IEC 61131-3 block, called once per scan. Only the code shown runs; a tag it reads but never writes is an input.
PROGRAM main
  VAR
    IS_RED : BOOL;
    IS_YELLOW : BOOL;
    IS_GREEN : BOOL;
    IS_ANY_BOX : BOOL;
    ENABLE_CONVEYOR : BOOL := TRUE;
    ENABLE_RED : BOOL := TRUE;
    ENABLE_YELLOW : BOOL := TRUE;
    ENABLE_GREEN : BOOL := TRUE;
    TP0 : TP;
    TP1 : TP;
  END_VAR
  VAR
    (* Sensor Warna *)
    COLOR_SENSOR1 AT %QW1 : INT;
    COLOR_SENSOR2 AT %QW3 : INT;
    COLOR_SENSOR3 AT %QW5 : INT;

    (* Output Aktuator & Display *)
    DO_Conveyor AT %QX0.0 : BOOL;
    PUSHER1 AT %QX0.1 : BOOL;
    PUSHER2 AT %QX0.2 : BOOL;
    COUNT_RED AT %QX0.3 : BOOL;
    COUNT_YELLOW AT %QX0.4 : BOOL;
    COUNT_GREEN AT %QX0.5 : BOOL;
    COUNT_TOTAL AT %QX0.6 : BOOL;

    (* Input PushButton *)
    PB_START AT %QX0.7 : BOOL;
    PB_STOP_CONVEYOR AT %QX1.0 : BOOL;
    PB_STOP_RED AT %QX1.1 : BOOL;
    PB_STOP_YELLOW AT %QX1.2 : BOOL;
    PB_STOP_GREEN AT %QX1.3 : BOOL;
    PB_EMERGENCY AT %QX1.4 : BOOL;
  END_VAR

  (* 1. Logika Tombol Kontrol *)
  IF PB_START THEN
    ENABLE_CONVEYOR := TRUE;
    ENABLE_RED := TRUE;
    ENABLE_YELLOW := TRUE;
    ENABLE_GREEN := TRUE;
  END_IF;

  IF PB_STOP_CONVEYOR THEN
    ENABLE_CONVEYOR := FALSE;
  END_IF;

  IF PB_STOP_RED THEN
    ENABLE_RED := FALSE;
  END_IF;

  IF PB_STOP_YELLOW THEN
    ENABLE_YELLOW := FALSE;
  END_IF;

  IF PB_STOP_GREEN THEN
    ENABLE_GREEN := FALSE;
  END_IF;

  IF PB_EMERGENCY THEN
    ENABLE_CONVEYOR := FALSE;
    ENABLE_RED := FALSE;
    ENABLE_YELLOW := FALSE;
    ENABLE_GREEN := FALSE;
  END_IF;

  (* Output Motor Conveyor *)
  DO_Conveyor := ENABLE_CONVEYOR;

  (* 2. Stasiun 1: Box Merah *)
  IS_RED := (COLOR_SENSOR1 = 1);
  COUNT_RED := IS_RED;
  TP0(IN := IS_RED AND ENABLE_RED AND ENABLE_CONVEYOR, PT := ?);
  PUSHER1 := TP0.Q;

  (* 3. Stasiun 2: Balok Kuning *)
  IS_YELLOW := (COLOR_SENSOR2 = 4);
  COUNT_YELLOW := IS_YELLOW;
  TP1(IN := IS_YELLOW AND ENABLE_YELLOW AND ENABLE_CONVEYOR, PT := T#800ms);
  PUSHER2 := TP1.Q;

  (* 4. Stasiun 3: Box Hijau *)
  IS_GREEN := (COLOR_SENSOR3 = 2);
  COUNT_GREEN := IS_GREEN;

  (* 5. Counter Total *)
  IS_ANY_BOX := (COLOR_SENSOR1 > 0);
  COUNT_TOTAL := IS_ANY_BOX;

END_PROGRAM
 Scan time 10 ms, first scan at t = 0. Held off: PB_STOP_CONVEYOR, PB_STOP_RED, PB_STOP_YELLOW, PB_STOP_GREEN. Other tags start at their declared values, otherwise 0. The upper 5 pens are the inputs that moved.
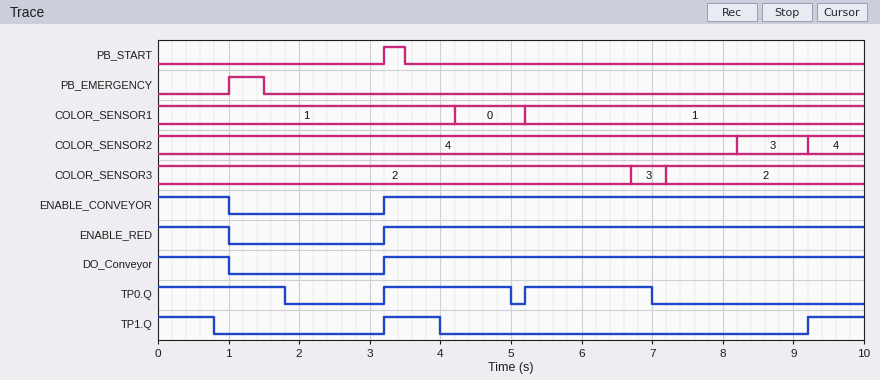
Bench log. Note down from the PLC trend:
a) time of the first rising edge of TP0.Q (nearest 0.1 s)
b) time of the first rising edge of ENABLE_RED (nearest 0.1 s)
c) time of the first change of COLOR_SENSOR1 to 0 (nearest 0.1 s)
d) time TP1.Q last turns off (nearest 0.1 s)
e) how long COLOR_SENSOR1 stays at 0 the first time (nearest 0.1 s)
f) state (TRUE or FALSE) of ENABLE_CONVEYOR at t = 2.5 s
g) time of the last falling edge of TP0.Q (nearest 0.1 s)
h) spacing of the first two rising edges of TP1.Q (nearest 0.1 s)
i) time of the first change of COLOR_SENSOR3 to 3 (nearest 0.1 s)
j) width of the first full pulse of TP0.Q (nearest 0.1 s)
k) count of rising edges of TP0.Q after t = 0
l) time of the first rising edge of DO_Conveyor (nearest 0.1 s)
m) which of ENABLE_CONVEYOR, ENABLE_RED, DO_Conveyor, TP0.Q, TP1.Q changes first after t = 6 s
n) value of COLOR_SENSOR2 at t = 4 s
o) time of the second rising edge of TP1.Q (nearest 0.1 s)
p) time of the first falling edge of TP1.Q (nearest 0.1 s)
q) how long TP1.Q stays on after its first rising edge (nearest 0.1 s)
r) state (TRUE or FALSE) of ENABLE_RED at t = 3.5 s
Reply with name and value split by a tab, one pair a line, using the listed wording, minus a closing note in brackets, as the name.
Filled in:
time of the first rising edge of TP0.Q	3.2 s
time of the first rising edge of ENABLE_RED	3.2 s
time of the first change of COLOR_SENSOR1 to 0	4.2 s
time TP1.Q last turns off	4.0 s
how long COLOR_SENSOR1 stays at 0 the first time	1.0 s
state (TRUE or FALSE) of ENABLE_CONVEYOR at t = 2.5 s	FALSE
time of the last falling edge of TP0.Q	7.0 s
spacing of the first two rising edges of TP1.Q	6.0 s
time of the first change of COLOR_SENSOR3 to 3	6.7 s
width of the first full pulse of TP0.Q	1.8 s
count of rising edges of TP0.Q after t = 0	2
time of the first rising edge of DO_Conveyor	3.2 s
which of ENABLE_CONVEYOR, ENABLE_RED, DO_Conveyor, TP0.Q, TP1.Q changes first after t = 6 s	TP0.Q
value of COLOR_SENSOR2 at t = 4 s	4
time of the second rising edge of TP1.Q	9.2 s
time of the first falling edge of TP1.Q	0.8 s
how long TP1.Q stays on after its first rising edge	0.8 s
state (TRUE or FALSE) of ENABLE_RED at t = 3.5 s	TRUE
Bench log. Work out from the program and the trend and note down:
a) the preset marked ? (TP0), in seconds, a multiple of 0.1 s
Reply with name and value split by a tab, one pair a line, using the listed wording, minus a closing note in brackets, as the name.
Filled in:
the preset marked ? (TP0), in seconds, a multiple of 0.1 s	1.8 s
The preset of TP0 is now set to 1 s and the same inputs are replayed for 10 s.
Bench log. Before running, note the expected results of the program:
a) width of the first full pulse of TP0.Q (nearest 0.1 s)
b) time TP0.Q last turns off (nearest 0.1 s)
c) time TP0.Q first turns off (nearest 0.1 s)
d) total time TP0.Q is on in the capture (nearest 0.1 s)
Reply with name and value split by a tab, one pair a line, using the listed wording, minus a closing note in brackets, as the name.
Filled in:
width of the first full pulse of TP0.Q	1.0 s
time TP0.Q last turns off	6.2 s
time TP0.Q first turns off	1.0 s
total time TP0.Q is on in the capture	3.0 s
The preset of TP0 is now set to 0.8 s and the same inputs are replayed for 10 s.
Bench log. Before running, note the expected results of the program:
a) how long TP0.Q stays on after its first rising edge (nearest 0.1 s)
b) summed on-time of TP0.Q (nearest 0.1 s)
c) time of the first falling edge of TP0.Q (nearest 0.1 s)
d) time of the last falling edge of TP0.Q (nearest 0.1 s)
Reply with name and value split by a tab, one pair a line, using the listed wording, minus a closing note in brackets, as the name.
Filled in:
how long TP0.Q stays on after its first rising edge	0.8 s
summed on-time of TP0.Q	2.4 s
time of the first falling edge of TP0.Q	0.8 s
time of the last falling edge of TP0.Q	6.0 s
